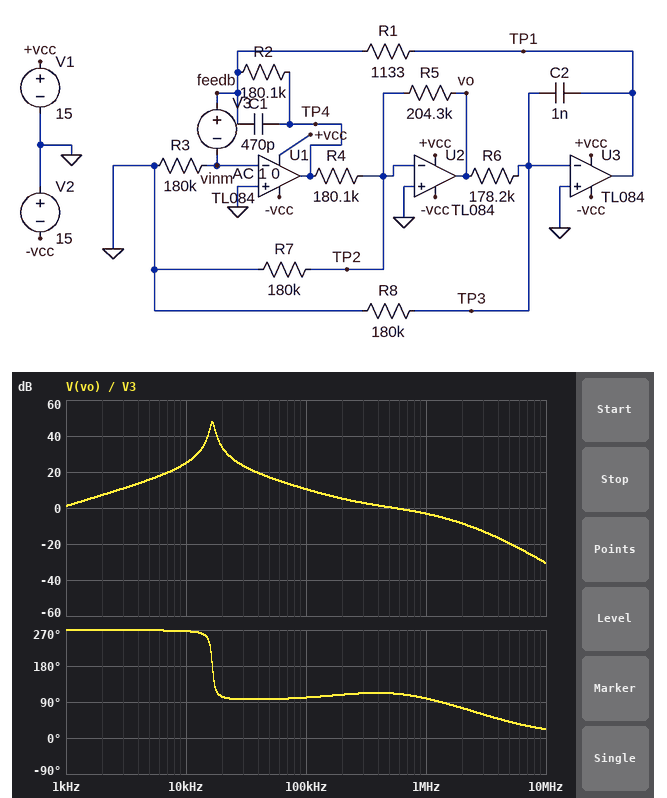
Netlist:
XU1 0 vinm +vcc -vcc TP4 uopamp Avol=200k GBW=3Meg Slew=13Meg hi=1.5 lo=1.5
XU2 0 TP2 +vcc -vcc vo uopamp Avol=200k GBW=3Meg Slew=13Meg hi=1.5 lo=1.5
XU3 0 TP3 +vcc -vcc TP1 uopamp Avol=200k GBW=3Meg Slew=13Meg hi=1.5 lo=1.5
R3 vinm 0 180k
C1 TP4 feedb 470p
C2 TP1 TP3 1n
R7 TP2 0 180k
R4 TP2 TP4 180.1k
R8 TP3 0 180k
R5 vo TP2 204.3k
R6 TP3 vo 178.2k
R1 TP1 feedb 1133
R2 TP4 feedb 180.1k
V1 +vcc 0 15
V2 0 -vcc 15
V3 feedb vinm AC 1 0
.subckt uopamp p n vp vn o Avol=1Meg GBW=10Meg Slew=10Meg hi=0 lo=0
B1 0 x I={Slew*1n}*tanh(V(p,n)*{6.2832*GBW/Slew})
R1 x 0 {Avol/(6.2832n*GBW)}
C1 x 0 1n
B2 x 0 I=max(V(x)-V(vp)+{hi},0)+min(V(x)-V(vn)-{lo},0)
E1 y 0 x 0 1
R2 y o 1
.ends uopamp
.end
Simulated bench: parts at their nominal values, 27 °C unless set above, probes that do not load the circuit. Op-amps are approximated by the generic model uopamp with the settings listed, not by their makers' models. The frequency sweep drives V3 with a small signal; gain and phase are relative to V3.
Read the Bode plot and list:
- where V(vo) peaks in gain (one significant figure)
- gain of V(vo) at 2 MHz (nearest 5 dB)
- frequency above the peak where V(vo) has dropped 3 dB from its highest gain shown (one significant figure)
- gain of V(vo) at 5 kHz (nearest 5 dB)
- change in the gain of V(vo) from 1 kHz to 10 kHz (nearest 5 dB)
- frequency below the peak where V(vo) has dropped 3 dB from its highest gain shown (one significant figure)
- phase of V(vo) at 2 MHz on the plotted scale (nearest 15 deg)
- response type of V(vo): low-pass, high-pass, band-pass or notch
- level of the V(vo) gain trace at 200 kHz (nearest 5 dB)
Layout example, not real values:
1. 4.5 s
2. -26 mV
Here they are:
1. 20 kHz
2. -10 dB
3. 20 kHz
4. 15 dB
5. 25 dB
6. 20 kHz
7. 75 deg
8. band-pass
9. 5 dB
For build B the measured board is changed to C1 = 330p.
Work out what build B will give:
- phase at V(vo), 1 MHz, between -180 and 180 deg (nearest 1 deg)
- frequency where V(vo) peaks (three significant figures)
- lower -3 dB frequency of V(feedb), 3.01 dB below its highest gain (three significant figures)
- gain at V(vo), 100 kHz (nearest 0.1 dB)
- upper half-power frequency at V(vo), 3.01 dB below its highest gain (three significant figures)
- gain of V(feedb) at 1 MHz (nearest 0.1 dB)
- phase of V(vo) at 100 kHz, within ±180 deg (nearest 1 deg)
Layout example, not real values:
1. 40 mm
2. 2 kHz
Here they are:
1. 93 deg
2. 19.4 kHz
3. 17.0 kHz
4. 13.1 dB
5. 20.3 kHz
6. -1.5 dB
7. 96 deg
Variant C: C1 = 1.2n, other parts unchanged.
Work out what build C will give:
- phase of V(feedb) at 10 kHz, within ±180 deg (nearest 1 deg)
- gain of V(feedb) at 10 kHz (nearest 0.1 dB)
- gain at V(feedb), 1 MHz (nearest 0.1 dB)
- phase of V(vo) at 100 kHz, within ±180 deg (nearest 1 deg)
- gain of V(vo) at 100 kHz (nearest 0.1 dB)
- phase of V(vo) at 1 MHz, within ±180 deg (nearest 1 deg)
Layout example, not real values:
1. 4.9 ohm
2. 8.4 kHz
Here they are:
1. -3 deg
2. 1.9 dB
3. -0.8 dB
4. 123 deg
5. 4.6 dB
6. 108 deg
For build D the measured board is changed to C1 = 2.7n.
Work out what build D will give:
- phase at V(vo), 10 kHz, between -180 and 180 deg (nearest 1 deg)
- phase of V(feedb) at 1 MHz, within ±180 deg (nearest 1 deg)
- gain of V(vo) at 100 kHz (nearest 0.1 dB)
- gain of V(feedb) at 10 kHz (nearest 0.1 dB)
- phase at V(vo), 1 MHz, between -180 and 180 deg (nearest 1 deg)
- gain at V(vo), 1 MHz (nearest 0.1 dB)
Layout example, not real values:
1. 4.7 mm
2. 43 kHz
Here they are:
1. 103 deg
2. -18 deg
3. 2.0 dB
4. -0.3 dB
5. 111 deg
6. -2.9 dB
